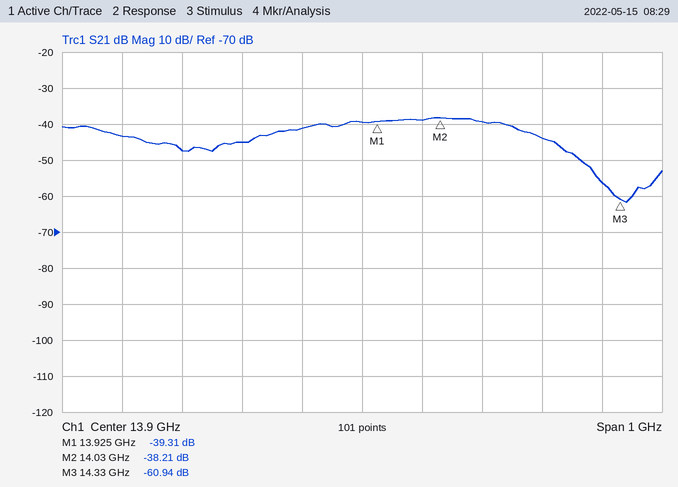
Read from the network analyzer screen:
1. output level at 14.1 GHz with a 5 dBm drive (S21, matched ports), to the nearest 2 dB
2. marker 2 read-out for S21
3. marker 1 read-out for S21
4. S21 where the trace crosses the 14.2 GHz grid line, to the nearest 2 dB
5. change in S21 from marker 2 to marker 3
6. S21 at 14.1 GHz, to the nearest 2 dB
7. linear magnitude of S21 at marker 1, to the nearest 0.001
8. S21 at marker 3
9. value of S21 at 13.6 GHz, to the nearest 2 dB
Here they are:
-34 dBm
-38.21 dB
-39.31 dB
-44 dB
-22.73 dB
-40 dB
0.011
-60.94 dB
-48 dB
